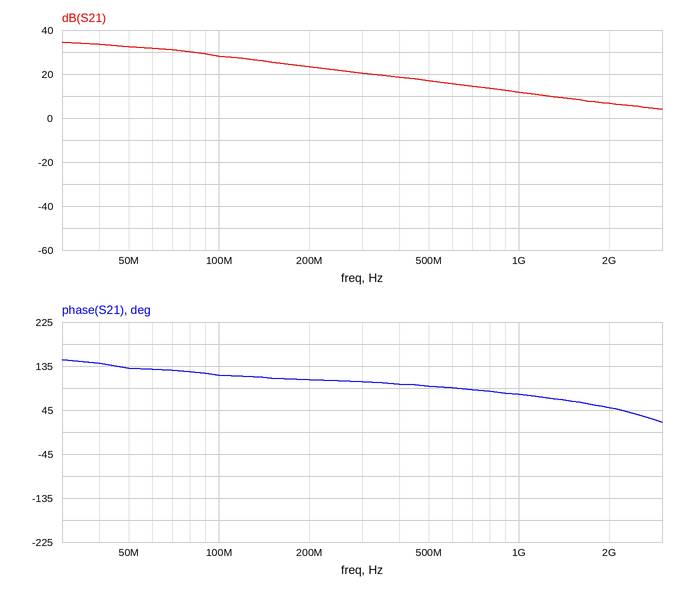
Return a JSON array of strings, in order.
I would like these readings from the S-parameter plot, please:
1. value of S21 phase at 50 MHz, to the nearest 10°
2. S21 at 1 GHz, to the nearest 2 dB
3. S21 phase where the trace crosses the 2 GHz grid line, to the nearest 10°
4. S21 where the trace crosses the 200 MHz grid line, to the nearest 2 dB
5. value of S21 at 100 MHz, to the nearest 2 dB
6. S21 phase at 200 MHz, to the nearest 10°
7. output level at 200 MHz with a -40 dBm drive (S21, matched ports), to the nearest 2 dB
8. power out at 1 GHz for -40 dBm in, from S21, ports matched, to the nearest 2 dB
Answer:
["130°", "12 dB", "50°", "24 dB", "28 dB", "110°", "-16 dBm", "-28 dBm"]
